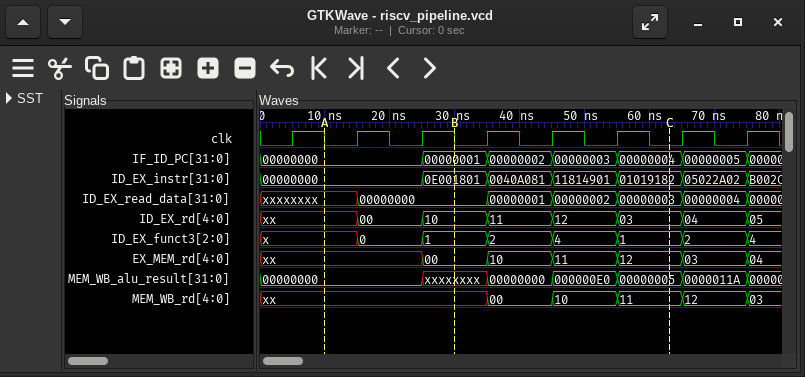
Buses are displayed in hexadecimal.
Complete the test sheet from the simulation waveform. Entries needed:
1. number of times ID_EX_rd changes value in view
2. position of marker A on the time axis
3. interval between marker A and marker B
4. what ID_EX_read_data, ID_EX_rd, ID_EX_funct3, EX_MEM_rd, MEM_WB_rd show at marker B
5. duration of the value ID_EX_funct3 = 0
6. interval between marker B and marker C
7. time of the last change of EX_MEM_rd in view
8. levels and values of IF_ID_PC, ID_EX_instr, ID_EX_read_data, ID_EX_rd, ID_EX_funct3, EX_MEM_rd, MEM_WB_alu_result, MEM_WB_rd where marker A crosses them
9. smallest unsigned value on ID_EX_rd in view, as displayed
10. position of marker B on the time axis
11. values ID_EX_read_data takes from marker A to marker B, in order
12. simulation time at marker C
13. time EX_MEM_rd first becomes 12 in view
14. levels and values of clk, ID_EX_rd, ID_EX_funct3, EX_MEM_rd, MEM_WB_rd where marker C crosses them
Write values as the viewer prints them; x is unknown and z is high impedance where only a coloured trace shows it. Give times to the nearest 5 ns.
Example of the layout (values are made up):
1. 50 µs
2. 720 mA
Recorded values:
1. 7
2. 10 ns
3. 20 ns
4. ID_EX_read_data=00000000, ID_EX_rd=10, ID_EX_funct3=1, EX_MEM_rd=00, MEM_WB_rd=xx
5. 10 ns
6. 35 ns
7. 75 ns
8. IF_ID_PC=00000000, ID_EX_instr=00000000, ID_EX_read_data=xxxxxxxx, ID_EX_rd=xx, ID_EX_funct3=x, EX_MEM_rd=xx, MEM_WB_alu_result=00000000, MEM_WB_rd=xx
9. 00
10. 30 ns
11. xxxxxxxx, 00000000
12. 65 ns
13. 55 ns
14. clk=0, ID_EX_rd=03, ID_EX_funct3=1, EX_MEM_rd=12, MEM_WB_rd=11
